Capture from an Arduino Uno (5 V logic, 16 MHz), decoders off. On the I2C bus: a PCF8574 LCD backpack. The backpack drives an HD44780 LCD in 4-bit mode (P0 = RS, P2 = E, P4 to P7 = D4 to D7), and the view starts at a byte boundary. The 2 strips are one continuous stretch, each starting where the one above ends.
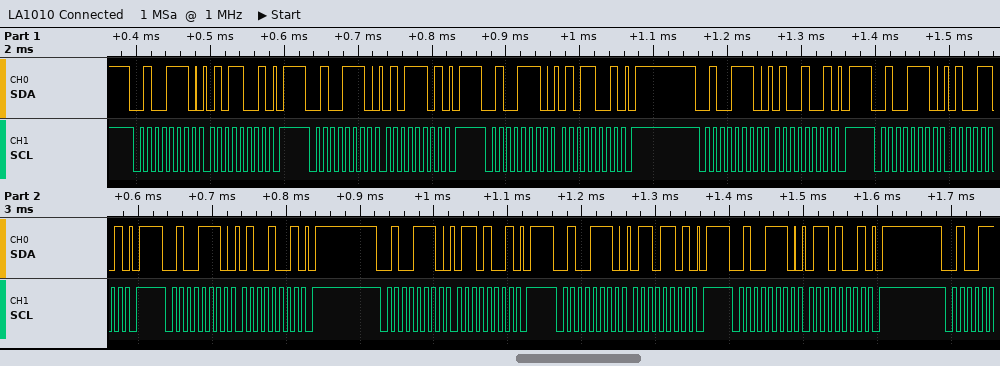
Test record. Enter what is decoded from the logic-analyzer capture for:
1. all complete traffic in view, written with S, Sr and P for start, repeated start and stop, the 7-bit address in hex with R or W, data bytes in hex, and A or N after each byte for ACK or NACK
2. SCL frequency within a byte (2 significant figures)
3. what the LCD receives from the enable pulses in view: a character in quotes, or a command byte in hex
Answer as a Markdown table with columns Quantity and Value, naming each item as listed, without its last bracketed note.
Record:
| Quantity | Value |
|---|---|
| all complete traffic in view, written with S, Sr and P for start, repeated start and stop, the 7-bit address in hex with R or W, data bytes in hex, and A or N after each byte for ACK or NACK | S 27W A 59 A P S 27W A 5D A P S 27W A 59 A P S 27W A 49 A P S 27W A 4D A P S 27W A 49 A P S 27W A 69 A P S 27W A 6D A P S 27W A 69 A P |
| SCL frequency within a byte | 100 kHz |
| what the LCD receives from the enable pulses in view: a character in quotes, or a command byte in hex | 'T' |
